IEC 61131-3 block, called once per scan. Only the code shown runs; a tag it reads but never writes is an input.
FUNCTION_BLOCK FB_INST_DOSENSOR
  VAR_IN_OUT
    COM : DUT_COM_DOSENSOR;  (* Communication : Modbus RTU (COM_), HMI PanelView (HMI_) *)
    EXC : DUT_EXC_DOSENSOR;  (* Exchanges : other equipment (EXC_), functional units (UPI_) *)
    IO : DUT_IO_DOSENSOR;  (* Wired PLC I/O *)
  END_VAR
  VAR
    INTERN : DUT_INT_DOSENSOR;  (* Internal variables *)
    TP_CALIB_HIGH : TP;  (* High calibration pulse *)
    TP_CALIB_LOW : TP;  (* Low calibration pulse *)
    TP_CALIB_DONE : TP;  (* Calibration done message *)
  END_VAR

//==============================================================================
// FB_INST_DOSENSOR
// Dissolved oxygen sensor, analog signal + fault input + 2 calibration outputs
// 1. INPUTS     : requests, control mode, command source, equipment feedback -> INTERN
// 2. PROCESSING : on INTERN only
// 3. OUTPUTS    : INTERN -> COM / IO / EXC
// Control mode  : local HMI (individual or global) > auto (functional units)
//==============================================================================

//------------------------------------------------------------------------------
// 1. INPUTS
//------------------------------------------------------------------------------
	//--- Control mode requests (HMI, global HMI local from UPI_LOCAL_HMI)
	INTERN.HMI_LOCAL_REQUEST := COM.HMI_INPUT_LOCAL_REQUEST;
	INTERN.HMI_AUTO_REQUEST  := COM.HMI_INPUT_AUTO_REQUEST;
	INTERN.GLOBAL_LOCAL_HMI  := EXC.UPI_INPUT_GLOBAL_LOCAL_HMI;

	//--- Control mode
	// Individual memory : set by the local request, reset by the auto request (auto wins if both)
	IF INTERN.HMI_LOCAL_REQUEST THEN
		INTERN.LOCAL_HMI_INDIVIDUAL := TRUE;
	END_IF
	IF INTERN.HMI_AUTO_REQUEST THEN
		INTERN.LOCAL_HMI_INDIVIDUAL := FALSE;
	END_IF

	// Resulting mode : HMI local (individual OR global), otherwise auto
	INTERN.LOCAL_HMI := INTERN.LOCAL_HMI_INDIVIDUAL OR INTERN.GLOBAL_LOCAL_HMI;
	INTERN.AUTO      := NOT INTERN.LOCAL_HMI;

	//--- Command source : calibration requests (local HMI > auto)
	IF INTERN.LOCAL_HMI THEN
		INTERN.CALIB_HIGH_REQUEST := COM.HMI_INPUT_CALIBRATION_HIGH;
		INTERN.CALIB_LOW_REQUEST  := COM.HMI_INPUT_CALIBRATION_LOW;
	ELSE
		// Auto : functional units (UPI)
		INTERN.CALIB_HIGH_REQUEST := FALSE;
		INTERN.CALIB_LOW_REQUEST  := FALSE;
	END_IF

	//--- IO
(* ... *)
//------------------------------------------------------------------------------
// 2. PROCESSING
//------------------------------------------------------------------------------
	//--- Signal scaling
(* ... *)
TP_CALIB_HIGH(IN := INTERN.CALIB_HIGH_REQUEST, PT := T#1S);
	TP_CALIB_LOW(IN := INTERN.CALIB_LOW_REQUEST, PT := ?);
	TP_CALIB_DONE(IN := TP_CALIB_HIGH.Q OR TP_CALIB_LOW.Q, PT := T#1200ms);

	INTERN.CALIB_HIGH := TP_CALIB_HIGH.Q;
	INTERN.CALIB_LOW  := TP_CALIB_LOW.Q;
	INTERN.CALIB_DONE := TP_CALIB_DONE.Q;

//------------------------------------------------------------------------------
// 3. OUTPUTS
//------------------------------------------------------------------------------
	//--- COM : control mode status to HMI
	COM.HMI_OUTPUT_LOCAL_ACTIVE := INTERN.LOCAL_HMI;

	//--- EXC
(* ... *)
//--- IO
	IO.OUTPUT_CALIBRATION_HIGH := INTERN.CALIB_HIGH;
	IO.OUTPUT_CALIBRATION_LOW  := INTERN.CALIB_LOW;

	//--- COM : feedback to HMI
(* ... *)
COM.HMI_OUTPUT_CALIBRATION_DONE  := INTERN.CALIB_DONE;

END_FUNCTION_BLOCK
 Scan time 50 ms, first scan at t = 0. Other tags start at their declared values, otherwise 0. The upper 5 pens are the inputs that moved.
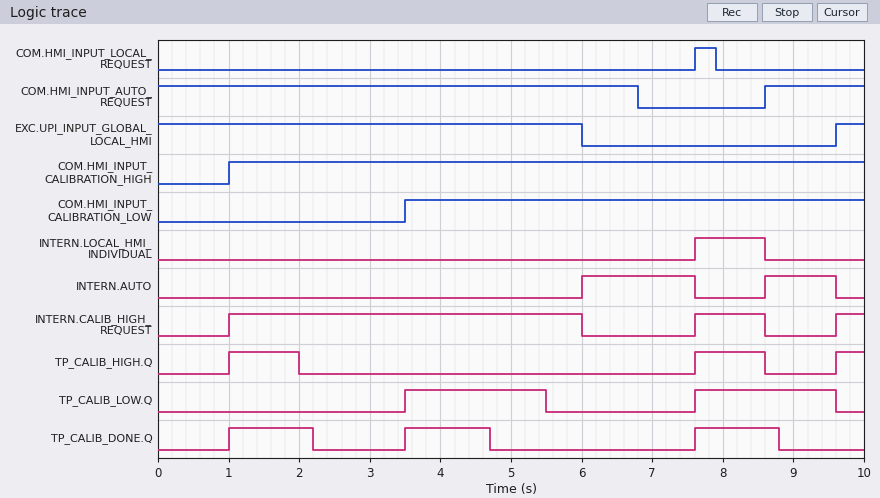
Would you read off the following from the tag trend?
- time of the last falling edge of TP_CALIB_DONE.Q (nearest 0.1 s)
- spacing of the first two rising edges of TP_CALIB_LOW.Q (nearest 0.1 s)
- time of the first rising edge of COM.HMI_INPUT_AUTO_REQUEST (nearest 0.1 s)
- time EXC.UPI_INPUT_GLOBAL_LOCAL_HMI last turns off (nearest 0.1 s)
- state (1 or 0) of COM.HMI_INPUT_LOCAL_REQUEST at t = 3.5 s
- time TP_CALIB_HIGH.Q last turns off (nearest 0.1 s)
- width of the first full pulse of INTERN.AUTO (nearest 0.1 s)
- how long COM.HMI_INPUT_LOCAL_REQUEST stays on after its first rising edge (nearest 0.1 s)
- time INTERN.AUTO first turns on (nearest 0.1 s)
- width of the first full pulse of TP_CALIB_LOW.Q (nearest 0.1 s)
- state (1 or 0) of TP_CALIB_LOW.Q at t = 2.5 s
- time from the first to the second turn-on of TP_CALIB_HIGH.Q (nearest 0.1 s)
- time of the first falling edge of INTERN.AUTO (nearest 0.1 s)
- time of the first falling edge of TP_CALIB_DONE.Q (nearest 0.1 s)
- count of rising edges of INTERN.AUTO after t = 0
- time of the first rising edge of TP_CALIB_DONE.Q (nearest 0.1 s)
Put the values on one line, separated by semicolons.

8.8 s; 4.1 s; 8.6 s; 6.0 s; 0; 8.6 s; 1.6 s; 0.3 s; 6.0 s; 2.0 s; 0; 6.6 s; 7.6 s; 2.2 s; 2; 1.0 s
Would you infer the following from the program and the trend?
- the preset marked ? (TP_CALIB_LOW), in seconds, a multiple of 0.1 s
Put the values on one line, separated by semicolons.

2.0 s
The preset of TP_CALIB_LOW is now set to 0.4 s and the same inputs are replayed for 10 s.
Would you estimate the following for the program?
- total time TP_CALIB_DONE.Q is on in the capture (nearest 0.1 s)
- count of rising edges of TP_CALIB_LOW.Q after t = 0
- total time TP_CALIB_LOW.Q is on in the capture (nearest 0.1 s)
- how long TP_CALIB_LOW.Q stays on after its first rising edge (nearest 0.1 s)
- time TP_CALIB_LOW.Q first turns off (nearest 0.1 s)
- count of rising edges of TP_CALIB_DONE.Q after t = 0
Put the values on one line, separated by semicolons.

4.0 s; 3; 1.2 s; 0.4 s; 3.9 s; 4
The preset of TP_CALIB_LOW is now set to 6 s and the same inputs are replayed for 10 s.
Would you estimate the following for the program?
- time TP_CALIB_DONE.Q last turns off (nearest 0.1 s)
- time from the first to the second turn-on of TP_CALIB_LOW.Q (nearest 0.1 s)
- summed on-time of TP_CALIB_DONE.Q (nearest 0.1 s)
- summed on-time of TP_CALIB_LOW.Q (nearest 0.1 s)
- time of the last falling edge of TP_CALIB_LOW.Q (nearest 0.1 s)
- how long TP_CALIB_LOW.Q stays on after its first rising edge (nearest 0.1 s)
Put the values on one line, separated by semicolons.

4.7 s; 6.1 s; 2.8 s; 6.4 s; 9.5 s; 6.0 s
